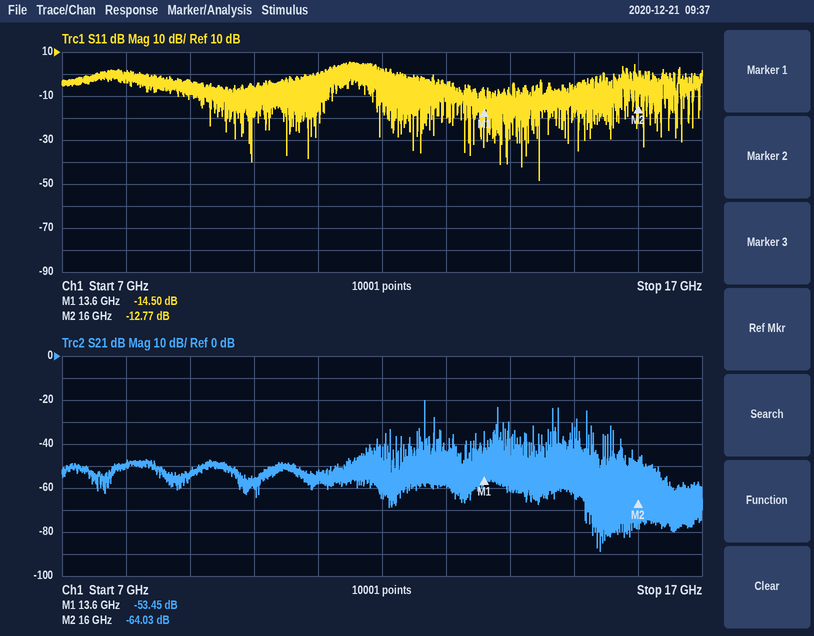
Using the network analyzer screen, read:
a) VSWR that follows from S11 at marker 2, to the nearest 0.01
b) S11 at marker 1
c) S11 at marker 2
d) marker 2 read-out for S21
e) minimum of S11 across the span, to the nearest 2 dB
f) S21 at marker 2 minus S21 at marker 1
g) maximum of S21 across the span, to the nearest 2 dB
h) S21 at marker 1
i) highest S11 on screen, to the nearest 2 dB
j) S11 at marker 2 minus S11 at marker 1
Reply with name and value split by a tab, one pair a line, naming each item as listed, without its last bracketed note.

VSWR that follows from S11 at marker 2, to the nearest 0.01	1.60
S11 at marker 1	-14.50 dB
S11 at marker 2	-12.77 dB
marker 2 read-out for S21	-64.03 dB
minimum of S11 across the span, to the nearest 2 dB	-48 dB
S21 at marker 2 minus S21 at marker 1	-10.58 dB
maximum of S21 across the span, to the nearest 2 dB	-20 dB
S21 at marker 1	-53.45 dB
highest S11 on screen, to the nearest 2 dB	6 dB
S11 at marker 2 minus S11 at marker 1	1.73 dB
